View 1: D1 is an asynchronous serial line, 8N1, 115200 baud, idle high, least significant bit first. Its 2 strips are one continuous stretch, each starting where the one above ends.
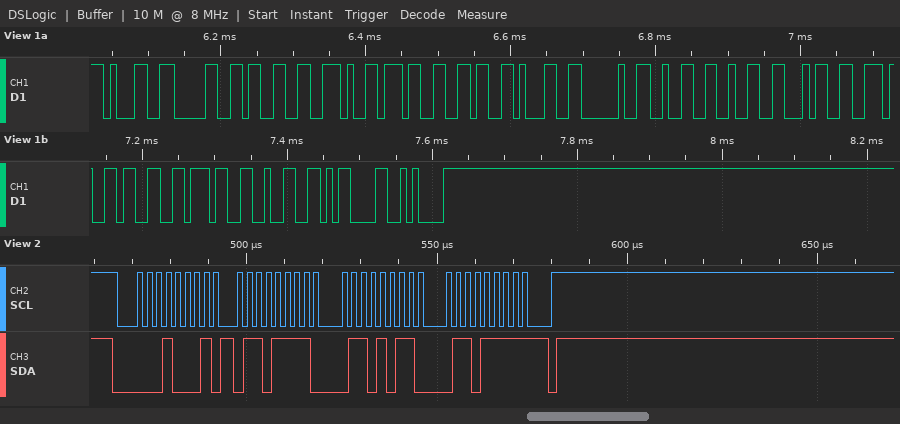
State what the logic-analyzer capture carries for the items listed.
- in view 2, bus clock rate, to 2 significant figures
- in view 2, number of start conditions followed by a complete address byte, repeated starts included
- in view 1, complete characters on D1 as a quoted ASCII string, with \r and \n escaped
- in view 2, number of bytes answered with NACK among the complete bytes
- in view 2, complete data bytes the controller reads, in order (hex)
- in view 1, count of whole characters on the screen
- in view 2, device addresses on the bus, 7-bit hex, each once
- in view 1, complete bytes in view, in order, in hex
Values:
400 kHz
1
"103.761 224.372\r\n"
1
6F 6B 6F
17
0x08
31 30 33 2E 37 36 31 20 32 32 34 2E 33 37 32 0D 0A
